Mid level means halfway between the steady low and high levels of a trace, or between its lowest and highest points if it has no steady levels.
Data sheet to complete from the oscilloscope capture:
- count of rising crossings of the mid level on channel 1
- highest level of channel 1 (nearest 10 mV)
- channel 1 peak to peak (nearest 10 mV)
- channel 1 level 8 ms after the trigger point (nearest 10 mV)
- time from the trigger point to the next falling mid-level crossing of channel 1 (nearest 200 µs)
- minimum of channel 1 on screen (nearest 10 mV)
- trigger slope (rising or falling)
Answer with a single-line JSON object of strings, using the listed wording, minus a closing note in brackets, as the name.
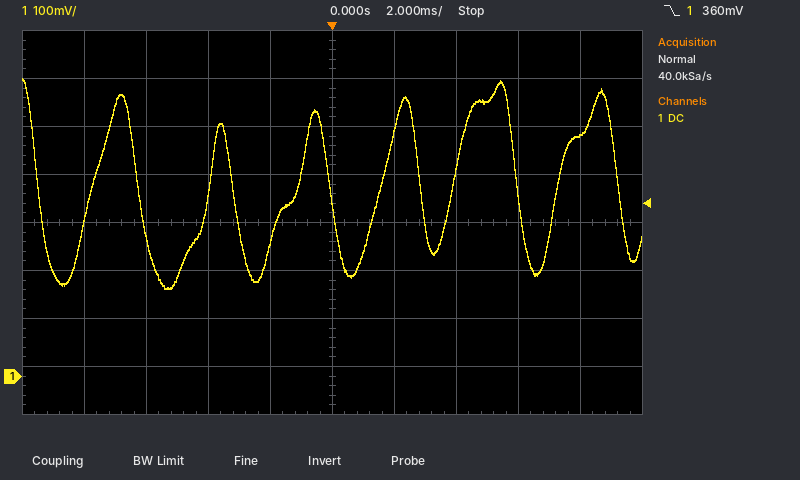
{"count of rising crossings of the mid level on channel 1": "6", "highest level of channel 1": "620 mV", "channel 1 peak to peak": "440 mV", "channel 1 level 8 ms after the trigger point": "500 mV", "time from the trigger point to the next falling mid-level crossing of channel 1": "2.8 ms", "minimum of channel 1 on screen": "180 mV", "trigger slope": "falling"}
